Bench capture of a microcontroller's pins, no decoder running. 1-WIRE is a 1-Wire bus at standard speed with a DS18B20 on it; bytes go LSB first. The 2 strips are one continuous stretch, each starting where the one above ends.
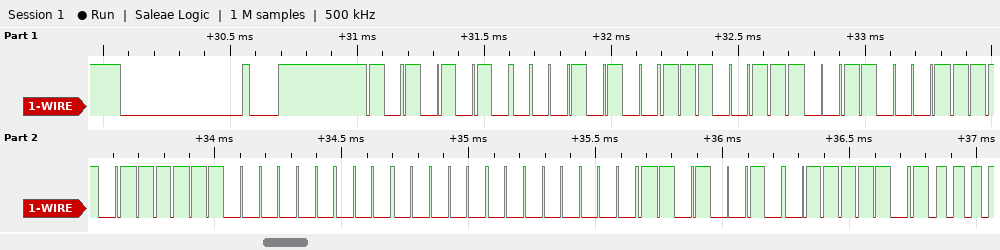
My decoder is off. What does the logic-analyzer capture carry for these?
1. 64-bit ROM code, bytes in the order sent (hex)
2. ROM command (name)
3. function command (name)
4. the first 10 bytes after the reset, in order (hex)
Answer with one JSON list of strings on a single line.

["28 E7 8C F7 03 00 00 4B", "Match ROM", "Read Scratchpad", "55 28 E7 8C F7 03 00 00 4B BE"]
